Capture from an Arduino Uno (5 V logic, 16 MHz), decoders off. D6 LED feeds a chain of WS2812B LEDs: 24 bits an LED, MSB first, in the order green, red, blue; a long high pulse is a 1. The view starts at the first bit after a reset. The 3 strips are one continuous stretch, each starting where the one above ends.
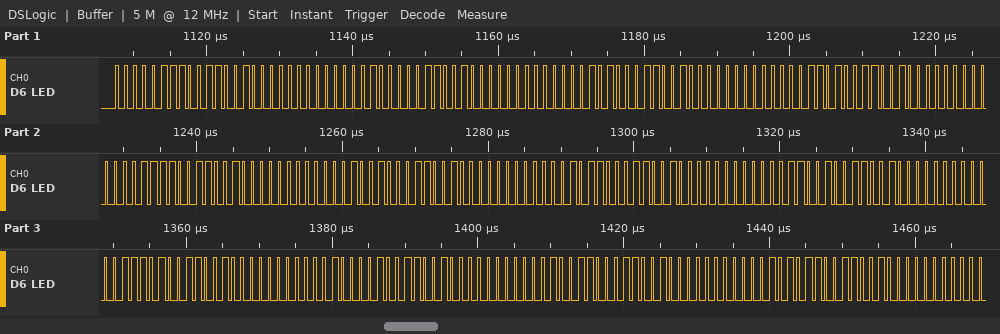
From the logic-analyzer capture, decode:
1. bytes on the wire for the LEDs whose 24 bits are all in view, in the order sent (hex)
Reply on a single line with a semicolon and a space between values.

07 32 00 08 32 00 0A 32 00 0D 32 00 0F 32 00 12 32 00 16 32 00 19 32 00 1D 32 00 21 32 00 26 32 00 2B 32 00
